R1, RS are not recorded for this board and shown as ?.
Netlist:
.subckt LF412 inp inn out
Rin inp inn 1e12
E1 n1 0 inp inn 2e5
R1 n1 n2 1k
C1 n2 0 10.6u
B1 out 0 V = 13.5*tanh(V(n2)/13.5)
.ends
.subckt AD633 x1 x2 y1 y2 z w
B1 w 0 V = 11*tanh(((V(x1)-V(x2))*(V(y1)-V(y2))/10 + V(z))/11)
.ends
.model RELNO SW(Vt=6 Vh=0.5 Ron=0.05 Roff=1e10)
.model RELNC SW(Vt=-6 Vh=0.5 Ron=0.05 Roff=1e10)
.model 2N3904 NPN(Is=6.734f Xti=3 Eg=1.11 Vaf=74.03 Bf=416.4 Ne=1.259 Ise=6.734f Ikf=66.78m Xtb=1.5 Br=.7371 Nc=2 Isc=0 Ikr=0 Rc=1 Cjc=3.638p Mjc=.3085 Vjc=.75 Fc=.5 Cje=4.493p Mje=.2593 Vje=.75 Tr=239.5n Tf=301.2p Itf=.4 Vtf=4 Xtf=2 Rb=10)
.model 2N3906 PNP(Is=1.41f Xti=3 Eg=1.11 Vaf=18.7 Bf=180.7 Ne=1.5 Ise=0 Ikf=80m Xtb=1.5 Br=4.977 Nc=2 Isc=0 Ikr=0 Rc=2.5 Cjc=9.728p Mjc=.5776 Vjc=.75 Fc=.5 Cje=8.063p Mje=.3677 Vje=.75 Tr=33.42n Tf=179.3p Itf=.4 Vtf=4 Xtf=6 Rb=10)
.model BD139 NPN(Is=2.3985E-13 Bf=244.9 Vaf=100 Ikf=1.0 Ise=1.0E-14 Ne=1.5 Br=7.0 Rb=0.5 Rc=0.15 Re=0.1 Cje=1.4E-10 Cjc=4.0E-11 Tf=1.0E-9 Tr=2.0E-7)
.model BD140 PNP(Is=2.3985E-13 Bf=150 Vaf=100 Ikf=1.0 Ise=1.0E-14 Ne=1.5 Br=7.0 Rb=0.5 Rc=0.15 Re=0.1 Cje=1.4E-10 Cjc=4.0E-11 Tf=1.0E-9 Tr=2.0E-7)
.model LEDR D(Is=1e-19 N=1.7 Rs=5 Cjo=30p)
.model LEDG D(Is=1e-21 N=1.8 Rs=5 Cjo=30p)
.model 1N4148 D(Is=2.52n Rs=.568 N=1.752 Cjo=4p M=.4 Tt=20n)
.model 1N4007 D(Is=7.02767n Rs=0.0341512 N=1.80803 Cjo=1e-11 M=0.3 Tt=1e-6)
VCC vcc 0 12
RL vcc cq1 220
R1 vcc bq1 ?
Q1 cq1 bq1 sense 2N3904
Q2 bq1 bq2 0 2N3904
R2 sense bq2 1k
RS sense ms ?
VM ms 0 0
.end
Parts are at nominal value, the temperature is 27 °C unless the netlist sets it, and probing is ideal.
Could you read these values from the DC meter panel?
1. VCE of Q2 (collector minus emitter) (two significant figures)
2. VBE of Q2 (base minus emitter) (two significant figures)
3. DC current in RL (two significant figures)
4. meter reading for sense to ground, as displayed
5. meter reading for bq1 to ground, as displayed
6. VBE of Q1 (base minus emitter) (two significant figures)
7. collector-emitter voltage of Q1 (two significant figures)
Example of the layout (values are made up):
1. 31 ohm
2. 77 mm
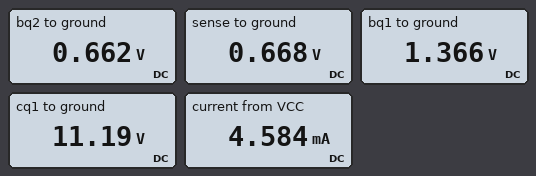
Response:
1. 1.4 V
2. 660 mV
3. 3.7 mA
4. 0.668 V
5. 1.366 V
6. 700 mV
7. 11 V
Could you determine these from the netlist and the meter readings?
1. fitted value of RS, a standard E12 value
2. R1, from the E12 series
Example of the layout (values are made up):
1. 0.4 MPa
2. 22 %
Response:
1. 180 Ω
2. 12 kΩ
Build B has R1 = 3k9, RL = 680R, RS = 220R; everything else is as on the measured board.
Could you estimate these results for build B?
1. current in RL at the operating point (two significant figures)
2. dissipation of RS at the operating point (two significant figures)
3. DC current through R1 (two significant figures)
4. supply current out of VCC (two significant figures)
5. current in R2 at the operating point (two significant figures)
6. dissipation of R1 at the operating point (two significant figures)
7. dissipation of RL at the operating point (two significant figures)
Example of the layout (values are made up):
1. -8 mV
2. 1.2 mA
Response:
1. 3.2 mA
2. 2.3 mW
3. 2.7 mA
4. 5.9 mA
5. 18 µA
6. 29 mW
7. 7.1 mW
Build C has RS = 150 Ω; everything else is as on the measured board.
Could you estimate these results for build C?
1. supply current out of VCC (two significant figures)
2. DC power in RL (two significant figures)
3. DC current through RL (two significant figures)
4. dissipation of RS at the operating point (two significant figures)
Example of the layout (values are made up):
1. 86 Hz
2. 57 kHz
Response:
1. 5.3 mA
2. 4.3 mW
3. 4.4 mA
4. 3.0 mW
